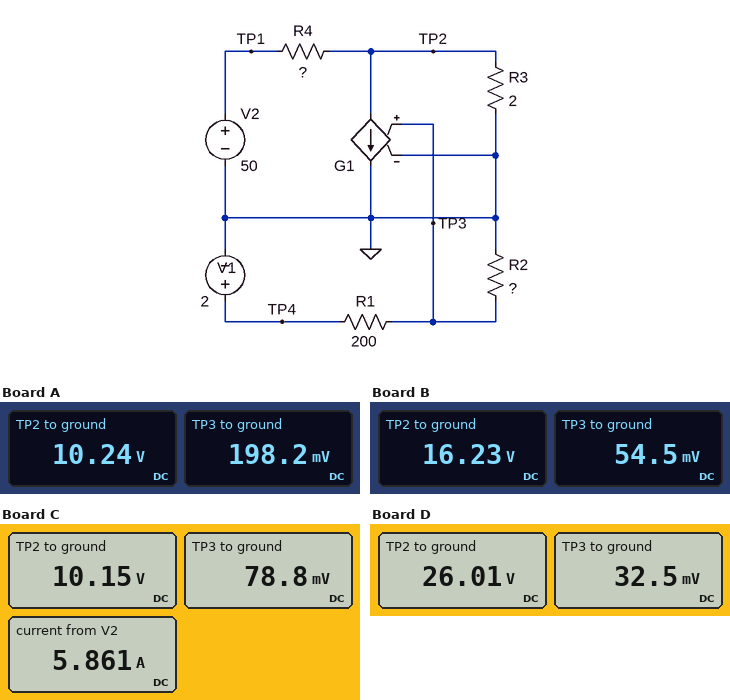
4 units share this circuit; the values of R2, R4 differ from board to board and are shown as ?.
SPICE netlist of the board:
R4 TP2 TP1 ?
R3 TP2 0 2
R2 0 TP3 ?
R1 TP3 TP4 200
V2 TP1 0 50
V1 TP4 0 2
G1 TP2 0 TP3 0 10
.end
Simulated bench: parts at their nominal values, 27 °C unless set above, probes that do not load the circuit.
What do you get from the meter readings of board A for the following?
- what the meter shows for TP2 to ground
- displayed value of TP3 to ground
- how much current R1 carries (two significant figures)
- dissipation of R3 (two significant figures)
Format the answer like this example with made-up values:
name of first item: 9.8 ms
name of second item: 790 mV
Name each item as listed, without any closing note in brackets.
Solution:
what the meter shows for TP2 to ground: 10.24 V
displayed value of TP3 to ground: 198.2 mV
how much current R1 carries: 9.0 mA
dissipation of R3: 52 W
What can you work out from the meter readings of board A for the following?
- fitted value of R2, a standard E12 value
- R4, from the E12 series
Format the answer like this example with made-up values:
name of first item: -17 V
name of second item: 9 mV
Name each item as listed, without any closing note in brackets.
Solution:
fitted value of R2, a standard E12 value: 22 Ω
R4, from the E12 series: 5.6 Ω
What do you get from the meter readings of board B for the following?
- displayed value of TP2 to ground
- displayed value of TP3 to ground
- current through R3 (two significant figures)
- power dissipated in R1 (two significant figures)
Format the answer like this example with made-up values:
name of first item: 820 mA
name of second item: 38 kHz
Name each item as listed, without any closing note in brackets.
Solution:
displayed value of TP2 to ground: 16.23 V
displayed value of TP3 to ground: 54.5 mV
current through R3: 8.1 A
power dissipated in R1: 19 mW
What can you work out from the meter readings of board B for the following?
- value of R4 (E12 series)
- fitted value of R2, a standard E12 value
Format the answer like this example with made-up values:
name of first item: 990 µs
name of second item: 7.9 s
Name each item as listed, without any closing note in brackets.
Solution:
value of R4: 3.9 Ω
fitted value of R2, a standard E12 value: 5.6 Ω
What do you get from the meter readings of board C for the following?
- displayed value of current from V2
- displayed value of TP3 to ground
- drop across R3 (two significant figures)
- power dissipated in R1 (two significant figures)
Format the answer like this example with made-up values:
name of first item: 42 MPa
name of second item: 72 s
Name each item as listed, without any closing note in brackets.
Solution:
displayed value of current from V2: 5.861 A
displayed value of TP3 to ground: 78.8 mV
drop across R3: 10 V
power dissipated in R1: 18 mW
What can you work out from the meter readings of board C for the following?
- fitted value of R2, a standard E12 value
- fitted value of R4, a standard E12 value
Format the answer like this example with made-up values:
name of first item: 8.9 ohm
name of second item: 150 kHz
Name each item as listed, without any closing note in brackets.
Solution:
fitted value of R2, a standard E12 value: 8.2 Ω
fitted value of R4, a standard E12 value: 6.8 Ω
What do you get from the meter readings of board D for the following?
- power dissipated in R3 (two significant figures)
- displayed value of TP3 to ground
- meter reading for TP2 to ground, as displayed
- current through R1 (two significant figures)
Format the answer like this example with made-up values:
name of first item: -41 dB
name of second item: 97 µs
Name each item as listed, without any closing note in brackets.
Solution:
power dissipated in R3: 340 W
displayed value of TP3 to ground: 32.5 mV
meter reading for TP2 to ground, as displayed: 26.01 V
current through R1: 9.8 mA
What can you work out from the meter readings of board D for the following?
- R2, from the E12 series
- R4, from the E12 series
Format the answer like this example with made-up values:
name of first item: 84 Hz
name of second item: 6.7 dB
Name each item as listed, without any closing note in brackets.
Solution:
R2, from the E12 series: 3.3 Ω
R4, from the E12 series: 1.8 Ω
